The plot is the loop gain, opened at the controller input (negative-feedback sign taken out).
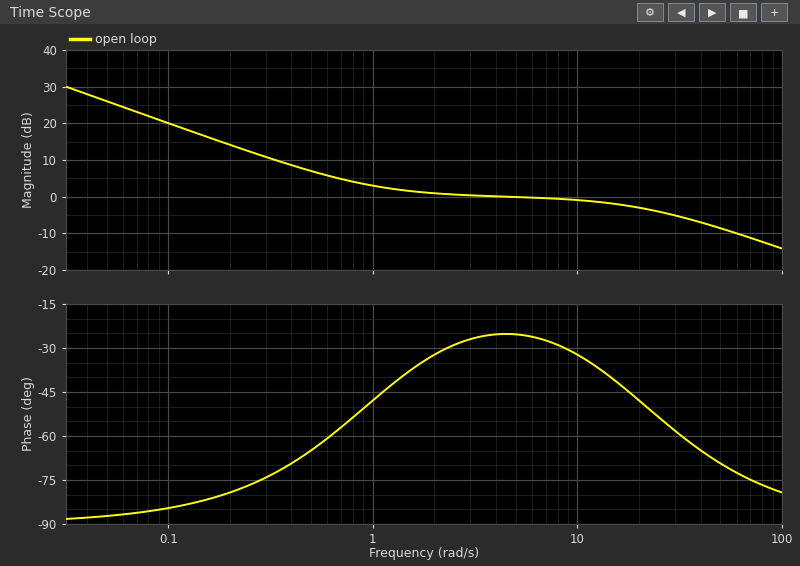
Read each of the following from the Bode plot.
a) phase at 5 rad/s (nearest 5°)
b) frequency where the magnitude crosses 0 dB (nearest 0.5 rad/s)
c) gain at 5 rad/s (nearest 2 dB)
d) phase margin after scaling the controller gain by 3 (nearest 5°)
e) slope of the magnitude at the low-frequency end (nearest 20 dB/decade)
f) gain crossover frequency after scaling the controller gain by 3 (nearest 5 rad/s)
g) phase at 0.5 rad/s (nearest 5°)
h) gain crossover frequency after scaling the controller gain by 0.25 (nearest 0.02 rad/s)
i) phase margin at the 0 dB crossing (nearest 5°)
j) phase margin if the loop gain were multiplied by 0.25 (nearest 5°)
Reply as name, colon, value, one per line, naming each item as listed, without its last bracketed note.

phase at 5 rad/s: -25°
frequency where the magnitude crosses 0 dB: 4.5 rad/s
gain at 5 rad/s: 0 dB
phase margin after scaling the controller gain by 3: 110°
slope of the magnitude at the low-frequency end: -20 dB/decade
gain crossover frequency after scaling the controller gain by 3: 55 rad/s
phase at 0.5 rad/s: -65°
gain crossover frequency after scaling the controller gain by 0.25: 0.26 rad/s
phase margin at the 0 dB crossing: 155°
phase margin if the loop gain were multiplied by 0.25: 105°
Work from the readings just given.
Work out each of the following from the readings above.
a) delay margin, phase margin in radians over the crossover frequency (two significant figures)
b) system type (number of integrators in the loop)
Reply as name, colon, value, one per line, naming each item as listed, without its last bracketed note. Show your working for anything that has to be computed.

delay margin, phase margin in radians over the crossover frequency: 155 × π / 180 / 4.5 = 0.60 s
system type: 1
